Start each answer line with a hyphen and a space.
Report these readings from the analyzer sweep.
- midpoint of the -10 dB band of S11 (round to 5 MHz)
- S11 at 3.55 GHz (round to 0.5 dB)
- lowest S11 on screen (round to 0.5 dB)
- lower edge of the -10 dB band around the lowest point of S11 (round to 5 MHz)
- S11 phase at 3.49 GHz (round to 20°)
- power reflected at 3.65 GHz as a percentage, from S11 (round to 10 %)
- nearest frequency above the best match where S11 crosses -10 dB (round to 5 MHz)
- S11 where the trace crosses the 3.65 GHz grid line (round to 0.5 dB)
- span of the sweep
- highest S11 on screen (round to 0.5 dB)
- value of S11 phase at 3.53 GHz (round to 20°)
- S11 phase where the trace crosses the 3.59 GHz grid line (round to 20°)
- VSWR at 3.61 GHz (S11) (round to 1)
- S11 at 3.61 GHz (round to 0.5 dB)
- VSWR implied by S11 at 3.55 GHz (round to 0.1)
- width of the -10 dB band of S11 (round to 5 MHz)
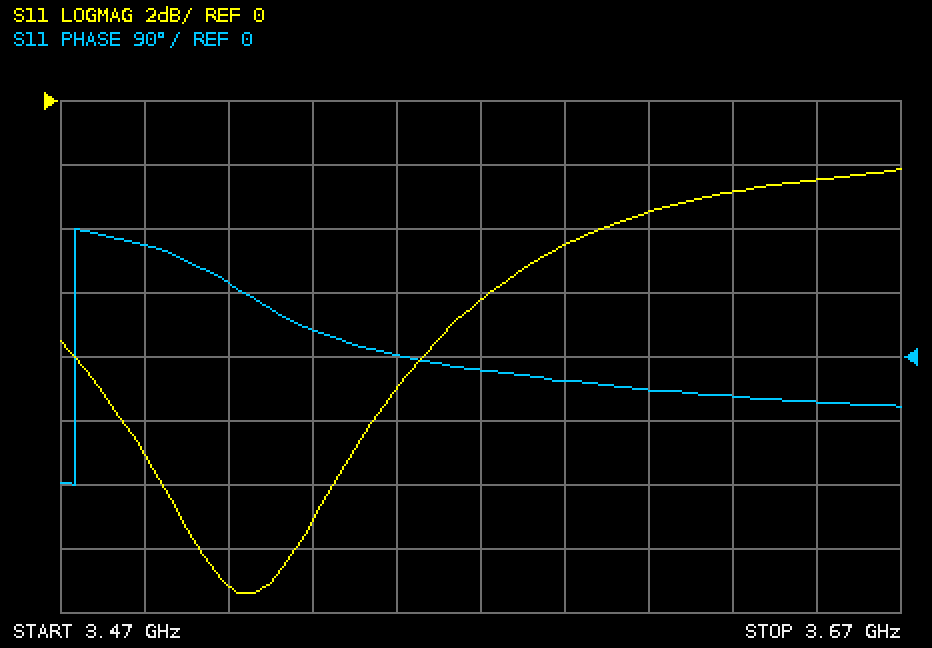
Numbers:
- 3.515 GHz
- -9.0 dB
- -15.5 dB
- 3.485 GHz
- 160°
- 60 %
- 3.545 GHz
- -2.5 dB
- 200 MHz
- -2.0 dB
- 40°
- -40°
- 5
- -3.5 dB
- 2.1
- 60 MHz
